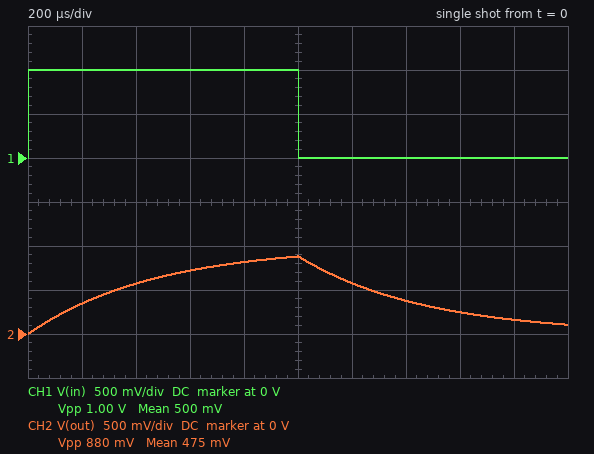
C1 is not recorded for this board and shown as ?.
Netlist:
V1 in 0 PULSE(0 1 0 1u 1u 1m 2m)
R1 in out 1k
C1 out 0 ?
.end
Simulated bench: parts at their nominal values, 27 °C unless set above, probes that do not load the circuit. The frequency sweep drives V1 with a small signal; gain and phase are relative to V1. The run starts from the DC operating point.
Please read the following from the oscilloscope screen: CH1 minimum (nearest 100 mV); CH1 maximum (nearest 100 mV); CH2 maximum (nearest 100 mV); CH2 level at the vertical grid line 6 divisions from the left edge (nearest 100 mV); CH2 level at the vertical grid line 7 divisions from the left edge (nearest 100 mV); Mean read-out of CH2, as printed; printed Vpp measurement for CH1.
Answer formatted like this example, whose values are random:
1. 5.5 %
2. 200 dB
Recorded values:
1. 0 V
2. 1.0 V
3. 900 mV
4. 600 mV
5. 400 mV
6. 475 mV
7. 1.00 V
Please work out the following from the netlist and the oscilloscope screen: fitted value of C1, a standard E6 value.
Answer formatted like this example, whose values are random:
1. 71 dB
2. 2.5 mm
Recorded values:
1. 470 nF
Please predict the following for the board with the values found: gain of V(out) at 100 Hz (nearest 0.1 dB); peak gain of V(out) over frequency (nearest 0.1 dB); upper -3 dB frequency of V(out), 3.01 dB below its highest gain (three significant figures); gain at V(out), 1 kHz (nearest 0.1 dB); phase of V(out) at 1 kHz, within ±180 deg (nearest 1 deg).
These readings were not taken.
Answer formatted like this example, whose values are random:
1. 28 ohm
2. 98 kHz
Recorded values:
1. -0.4 dB
2. 0 dB
3. 339 Hz
4. -9.9 dB
5. -71 deg
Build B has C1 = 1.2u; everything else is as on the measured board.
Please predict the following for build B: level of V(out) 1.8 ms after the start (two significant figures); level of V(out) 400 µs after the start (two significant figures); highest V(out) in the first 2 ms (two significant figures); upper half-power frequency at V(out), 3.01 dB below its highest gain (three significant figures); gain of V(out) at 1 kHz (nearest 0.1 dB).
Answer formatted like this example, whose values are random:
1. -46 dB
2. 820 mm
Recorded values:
1. 290 mV
2. 280 mV
3. 570 mV
4. 133 Hz
5. -17.6 dB
